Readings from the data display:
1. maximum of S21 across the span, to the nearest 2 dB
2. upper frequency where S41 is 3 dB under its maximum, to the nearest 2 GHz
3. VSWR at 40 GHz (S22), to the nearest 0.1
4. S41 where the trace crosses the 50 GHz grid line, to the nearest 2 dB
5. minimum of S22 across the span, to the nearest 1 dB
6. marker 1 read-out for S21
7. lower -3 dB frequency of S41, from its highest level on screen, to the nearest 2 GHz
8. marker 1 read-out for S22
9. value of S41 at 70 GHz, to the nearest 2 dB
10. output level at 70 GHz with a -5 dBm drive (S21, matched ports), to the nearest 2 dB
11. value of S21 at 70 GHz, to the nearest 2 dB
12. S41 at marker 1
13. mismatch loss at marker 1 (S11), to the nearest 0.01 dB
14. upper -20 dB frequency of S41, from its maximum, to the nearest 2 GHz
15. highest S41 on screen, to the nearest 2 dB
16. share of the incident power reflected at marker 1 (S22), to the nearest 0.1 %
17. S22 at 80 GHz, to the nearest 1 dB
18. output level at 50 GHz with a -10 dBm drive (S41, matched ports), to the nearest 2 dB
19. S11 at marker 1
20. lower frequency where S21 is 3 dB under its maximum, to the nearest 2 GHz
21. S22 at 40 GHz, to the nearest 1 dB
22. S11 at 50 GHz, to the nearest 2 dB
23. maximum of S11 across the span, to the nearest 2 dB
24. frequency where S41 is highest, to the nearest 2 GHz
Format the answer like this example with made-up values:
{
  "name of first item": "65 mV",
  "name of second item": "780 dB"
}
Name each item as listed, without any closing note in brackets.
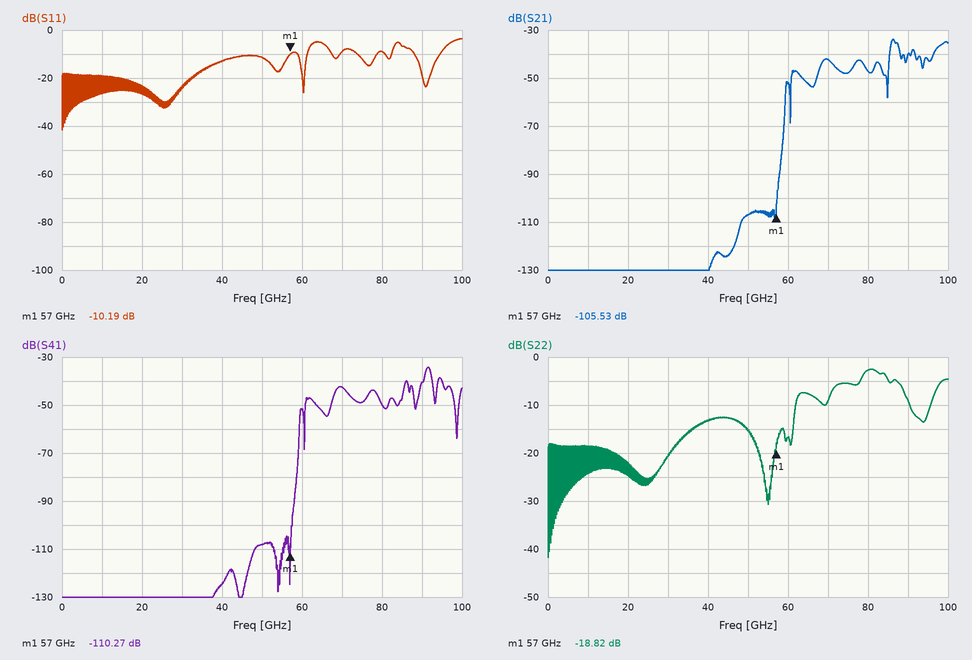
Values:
{
  "maximum of S21 across the span, to the nearest 2 dB": "-34 dB",
  "upper frequency where S41 is 3 dB under its maximum, to the nearest 2 GHz": "92 GHz",
  "VSWR at 40 GHz (S22), to the nearest 0.1": "1.6",
  "S41 where the trace crosses the 50 GHz grid line, to the nearest 2 dB": "-108 dB",
  "minimum of S22 across the span, to the nearest 1 dB": "-42 dB",
  "marker 1 read-out for S21": "-105.53 dB",
  "lower -3 dB frequency of S41, from its highest level on screen, to the nearest 2 GHz": "90 GHz",
  "marker 1 read-out for S22": "-18.82 dB",
  "value of S41 at 70 GHz, to the nearest 2 dB": "-42 dB",
  "output level at 70 GHz with a -5 dBm drive (S21, matched ports), to the nearest 2 dB": "-48 dBm",
  "value of S21 at 70 GHz, to the nearest 2 dB": "-42 dB",
  "S41 at marker 1": "-110.27 dB",
  "mismatch loss at marker 1 (S11), to the nearest 0.01 dB": "0.44 dB",
  "upper -20 dB frequency of S41, from its maximum, to the nearest 2 GHz": "98 GHz",
  "highest S41 on screen, to the nearest 2 dB": "-34 dB",
  "share of the incident power reflected at marker 1 (S22), to the nearest 0.1 %": "1.3 %",
  "S22 at 80 GHz, to the nearest 1 dB": "-3 dB",
  "output level at 50 GHz with a -10 dBm drive (S41, matched ports), to the nearest 2 dB": "-118 dBm",
  "S11 at marker 1": "-10.19 dB",
  "lower frequency where S21 is 3 dB under its maximum, to the nearest 2 GHz": "86 GHz",
  "S22 at 40 GHz, to the nearest 1 dB": "-13 dB",
  "S11 at 50 GHz, to the nearest 2 dB": "-12 dB",
  "maximum of S11 across the span, to the nearest 2 dB": "-4 dB",
  "frequency where S41 is highest, to the nearest 2 GHz": "92 GHz"
}
